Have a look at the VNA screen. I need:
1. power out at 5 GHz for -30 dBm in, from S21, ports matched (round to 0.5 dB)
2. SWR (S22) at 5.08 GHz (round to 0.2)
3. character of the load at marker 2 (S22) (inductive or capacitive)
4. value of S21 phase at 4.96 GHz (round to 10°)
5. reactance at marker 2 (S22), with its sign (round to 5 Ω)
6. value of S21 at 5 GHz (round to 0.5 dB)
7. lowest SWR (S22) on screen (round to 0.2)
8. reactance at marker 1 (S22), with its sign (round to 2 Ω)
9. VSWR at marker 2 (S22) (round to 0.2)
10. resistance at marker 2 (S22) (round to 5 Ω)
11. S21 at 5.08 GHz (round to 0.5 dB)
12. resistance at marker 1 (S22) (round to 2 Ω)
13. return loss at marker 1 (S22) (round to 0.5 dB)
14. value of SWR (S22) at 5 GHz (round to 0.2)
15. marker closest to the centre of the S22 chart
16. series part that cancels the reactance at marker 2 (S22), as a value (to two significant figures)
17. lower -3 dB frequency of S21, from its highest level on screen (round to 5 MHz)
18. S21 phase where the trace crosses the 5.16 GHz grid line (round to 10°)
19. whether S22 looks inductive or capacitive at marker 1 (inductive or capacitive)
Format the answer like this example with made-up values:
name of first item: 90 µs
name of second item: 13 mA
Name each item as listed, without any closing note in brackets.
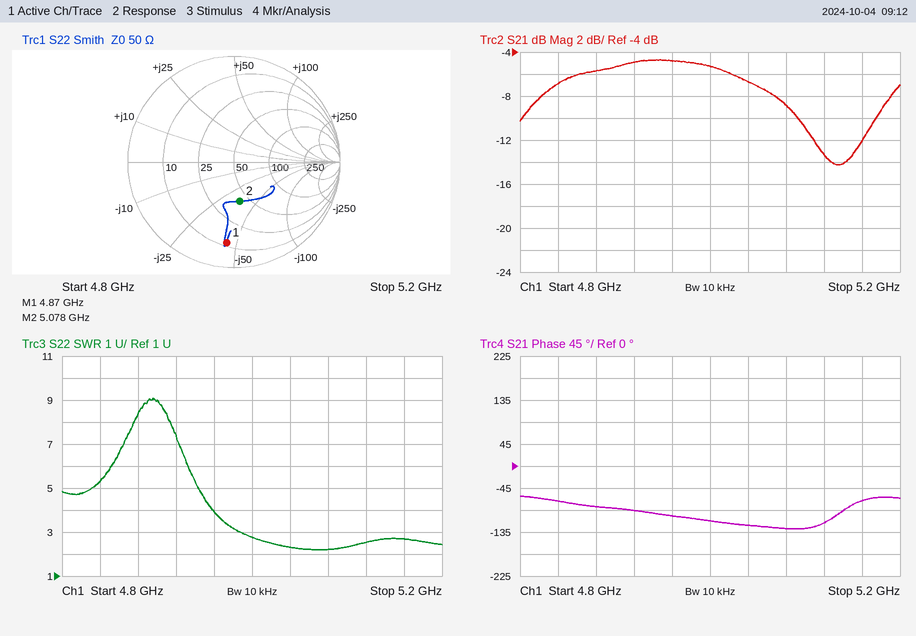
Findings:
power out at 5 GHz for -30 dBm in, from S21, ports matched: -35.5 dBm
SWR (S22) at 5.08 GHz: 2.2
character of the load at marker 2 (S22): capacitive
value of S21 phase at 4.96 GHz: -100°
reactance at marker 2 (S22), with its sign: -35 Ω
value of S21 at 5 GHz: -5.5 dB
lowest SWR (S22) on screen: 2.2
reactance at marker 1 (S22), with its sign: -44 Ω
VSWR at marker 2 (S22): 2.2
resistance at marker 2 (S22): 40 Ω
S21 at 5.08 GHz: -9.0 dB
resistance at marker 1 (S22): 12 Ω
return loss at marker 1 (S22): 2.5 dB
value of SWR (S22) at 5 GHz: 2.8
marker closest to the centre of the S22 chart: marker 2
series part that cancels the reactance at marker 2 (S22), as a value: 1.1 nH
lower -3 dB frequency of S21, from its highest level on screen: 4.825 GHz
S21 phase where the trace crosses the 5.16 GHz grid line: -70°
whether S22 looks inductive or capacitive at marker 1: capacitive
